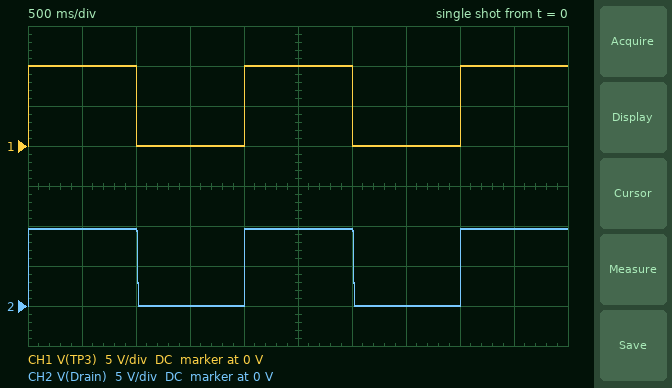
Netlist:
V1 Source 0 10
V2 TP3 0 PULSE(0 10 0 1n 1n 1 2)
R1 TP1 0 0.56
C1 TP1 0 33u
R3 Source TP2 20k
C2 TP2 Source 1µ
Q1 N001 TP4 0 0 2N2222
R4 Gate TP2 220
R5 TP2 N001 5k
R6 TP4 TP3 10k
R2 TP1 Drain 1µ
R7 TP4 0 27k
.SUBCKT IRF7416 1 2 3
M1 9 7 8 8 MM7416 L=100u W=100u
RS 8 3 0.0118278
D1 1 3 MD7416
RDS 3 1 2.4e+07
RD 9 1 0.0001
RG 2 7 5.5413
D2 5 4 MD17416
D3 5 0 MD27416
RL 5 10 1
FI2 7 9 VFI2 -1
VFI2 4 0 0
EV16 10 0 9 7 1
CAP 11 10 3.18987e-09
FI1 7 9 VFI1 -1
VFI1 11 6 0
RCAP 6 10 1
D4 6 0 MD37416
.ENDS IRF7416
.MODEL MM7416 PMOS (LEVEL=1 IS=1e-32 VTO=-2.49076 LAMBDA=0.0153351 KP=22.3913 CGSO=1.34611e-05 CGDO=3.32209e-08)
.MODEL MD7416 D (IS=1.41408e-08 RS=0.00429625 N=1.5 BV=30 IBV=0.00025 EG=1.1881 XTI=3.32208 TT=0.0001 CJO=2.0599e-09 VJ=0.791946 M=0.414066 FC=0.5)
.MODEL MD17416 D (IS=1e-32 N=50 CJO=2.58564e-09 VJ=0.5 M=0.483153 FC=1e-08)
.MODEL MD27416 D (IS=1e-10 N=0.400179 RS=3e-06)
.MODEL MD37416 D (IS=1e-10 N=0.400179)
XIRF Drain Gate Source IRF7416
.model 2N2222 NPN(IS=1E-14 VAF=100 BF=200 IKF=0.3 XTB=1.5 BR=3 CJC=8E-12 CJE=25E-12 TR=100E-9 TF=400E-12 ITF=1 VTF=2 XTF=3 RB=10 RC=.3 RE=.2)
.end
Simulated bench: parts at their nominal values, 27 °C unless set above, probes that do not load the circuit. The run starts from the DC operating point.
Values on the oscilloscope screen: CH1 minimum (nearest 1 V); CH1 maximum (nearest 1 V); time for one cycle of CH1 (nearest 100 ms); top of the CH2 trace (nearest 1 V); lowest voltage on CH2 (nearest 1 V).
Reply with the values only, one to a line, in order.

0 V
10 V
2.0 s
10 V
0 V
